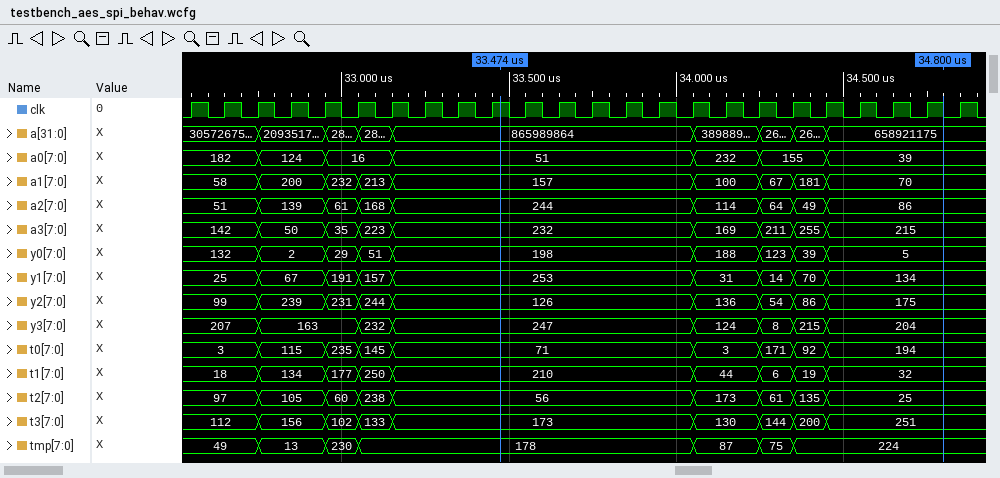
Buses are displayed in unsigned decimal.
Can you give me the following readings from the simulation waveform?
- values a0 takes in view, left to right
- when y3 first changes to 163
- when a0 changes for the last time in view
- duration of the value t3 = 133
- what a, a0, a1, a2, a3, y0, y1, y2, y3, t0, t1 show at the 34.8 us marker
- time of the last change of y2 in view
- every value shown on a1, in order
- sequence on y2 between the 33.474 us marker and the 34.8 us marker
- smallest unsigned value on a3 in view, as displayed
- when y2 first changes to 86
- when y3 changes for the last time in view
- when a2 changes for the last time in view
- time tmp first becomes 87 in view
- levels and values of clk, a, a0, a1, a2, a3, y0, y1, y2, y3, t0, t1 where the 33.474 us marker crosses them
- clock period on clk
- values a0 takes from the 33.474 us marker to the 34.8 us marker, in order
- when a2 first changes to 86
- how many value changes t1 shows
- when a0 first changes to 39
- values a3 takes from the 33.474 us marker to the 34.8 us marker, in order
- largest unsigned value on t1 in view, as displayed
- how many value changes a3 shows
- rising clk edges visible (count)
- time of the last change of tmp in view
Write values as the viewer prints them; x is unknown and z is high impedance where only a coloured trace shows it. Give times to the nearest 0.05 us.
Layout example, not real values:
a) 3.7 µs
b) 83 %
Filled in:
a) 182, 124, 16, 51, 232, 155, 39
b) 32.75 us
c) 34.45 us
d) 0.1 us
e) a=658921175, a0=39, a1=70, a2=86, a3=215, y0=5, y1=134, y2=175, y3=204, t0=194, t1=32
f) 34.45 us
g) 58, 200, 232, 213, 157, 100, 67, 181, 70
h) 126, 136, 54, 86, 175
i) 35
j) 34.35 us
k) 34.45 us
l) 34.45 us
m) 34.05 us
n) clk=1, a=865989864, a0=51, a1=157, a2=244, a3=232, y0=198, y1=253, y2=126, y3=247, t0=71, t1=210
o) 0.1 us
p) 51, 232, 155, 39
q) 34.45 us
r) 8
s) 34.45 us
t) 232, 169, 211, 255, 215
u) 250
v) 8
w) 24
x) 34.35 us
